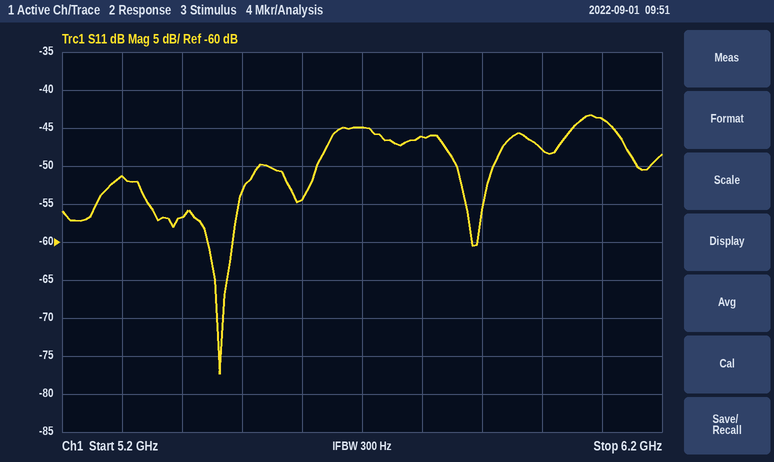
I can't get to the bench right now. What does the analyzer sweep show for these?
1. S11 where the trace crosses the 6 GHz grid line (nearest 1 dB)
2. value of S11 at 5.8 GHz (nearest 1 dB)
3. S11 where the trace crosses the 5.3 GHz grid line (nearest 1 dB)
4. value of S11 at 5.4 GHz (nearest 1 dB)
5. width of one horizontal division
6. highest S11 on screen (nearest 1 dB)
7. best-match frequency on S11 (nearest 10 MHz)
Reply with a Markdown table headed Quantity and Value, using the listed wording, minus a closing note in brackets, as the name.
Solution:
| Quantity | Value |
|---|---|
| S11 where the trace crosses the 6 GHz grid line | -48 dB |
| value of S11 at 5.8 GHz | -46 dB |
| S11 where the trace crosses the 5.3 GHz grid line | -51 dB |
| value of S11 at 5.4 GHz | -57 dB |
| width of one horizontal division | 100 MHz |
| highest S11 on screen | -43 dB |
| best-match frequency on S11 | 5.46 GHz |
